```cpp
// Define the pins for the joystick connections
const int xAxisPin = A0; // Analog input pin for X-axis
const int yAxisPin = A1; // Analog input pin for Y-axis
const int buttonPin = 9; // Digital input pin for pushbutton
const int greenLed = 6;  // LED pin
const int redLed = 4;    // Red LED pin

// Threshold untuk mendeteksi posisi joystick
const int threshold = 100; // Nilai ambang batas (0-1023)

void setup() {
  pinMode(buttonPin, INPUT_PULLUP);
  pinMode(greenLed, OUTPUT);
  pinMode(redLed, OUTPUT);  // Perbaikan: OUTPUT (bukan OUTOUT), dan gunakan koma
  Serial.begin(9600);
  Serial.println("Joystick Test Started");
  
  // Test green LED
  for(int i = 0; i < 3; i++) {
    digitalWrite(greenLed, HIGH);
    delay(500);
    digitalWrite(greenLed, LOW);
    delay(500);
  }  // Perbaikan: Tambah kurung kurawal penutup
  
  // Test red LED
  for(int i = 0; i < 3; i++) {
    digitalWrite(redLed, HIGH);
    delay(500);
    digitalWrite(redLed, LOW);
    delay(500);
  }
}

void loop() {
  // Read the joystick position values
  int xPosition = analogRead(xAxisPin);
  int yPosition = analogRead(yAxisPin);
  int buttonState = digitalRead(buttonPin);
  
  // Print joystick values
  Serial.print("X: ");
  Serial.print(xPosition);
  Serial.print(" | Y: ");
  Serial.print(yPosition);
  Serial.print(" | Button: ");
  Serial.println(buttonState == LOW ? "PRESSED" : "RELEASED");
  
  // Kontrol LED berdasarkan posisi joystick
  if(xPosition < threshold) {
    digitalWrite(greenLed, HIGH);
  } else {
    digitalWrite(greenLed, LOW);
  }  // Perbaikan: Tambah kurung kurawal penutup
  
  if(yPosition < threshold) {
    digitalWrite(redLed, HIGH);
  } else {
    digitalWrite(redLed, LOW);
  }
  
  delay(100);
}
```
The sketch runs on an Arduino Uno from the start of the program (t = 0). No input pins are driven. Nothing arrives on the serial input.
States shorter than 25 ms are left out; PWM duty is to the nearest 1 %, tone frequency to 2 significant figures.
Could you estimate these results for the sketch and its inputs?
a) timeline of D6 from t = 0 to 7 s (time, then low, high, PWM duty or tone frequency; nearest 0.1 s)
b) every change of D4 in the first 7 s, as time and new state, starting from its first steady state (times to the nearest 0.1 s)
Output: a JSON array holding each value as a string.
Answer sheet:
["0 s high; 0.5 s low; 1 s high; 1.5 s low; 2 s high; 2.5 s low; 6 s high", "0 s low; 3 s high; 3.5 s low; 4 s high; 4.5 s low; 5 s high; 5.5 s low; 6 s high"]
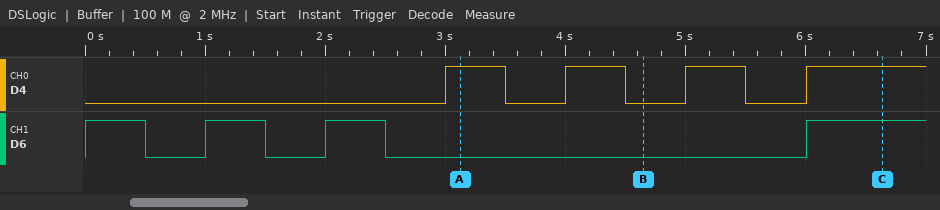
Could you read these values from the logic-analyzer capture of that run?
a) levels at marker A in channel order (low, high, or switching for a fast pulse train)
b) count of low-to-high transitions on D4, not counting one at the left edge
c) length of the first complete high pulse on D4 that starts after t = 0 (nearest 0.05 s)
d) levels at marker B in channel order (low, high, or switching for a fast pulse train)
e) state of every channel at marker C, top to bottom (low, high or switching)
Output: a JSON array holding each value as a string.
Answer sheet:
["D4 high, D6 low", "4", "0.50 s", "D4 low, D6 low", "D4 high, D6 high"]
